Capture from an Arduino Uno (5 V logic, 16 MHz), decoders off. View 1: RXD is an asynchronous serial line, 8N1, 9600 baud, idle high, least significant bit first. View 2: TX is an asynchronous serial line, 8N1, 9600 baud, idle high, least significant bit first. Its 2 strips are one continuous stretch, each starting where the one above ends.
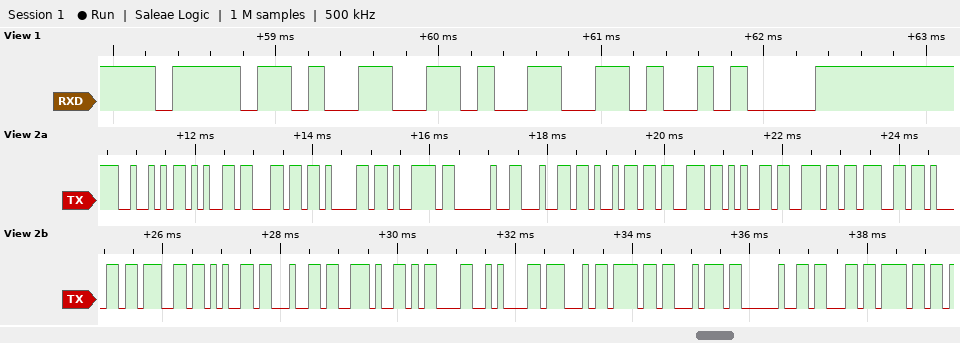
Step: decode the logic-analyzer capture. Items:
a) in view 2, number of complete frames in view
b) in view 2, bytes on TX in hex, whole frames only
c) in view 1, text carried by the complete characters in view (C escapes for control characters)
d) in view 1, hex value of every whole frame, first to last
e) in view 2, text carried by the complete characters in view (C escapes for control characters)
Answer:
25
52 65 6C 61 79 20 64 69 73 65 6E 67 61 67 65 64 2E 0D 0A 47 6F 74 20 63 6F
"off\n"
0x6F 0x66 0x66 0x0A
"Relay disengaged.\r\nGot co"
